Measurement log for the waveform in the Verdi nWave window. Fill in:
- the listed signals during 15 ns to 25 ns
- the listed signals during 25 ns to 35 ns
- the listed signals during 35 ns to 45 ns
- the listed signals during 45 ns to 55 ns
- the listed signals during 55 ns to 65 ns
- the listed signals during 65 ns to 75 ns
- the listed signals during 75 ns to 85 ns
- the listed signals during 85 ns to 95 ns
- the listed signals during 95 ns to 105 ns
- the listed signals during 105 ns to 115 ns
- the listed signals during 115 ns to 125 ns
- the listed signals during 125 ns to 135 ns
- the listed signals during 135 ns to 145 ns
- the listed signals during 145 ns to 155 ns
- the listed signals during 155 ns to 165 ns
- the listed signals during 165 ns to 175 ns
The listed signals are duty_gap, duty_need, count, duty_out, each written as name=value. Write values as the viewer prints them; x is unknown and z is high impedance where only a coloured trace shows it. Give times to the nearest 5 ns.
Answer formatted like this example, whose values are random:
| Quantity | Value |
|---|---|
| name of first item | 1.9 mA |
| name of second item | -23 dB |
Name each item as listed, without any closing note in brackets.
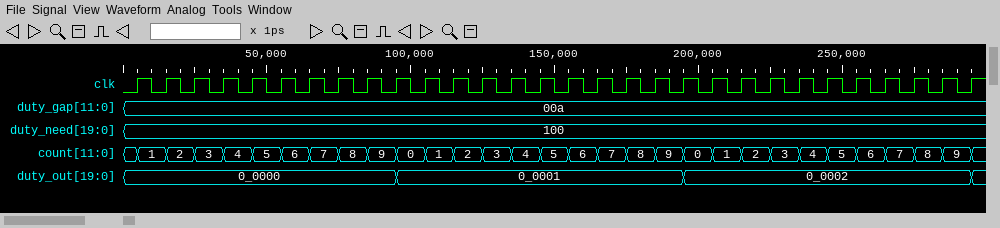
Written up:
| Quantity | Value |
|---|---|
| the listed signals during 15 ns to 25 ns | duty_gap=00a, duty_need=100, count=2, duty_out=0_0000 |
| the listed signals during 25 ns to 35 ns | duty_gap=00a, duty_need=100, count=3, duty_out=0_0000 |
| the listed signals during 35 ns to 45 ns | duty_gap=00a, duty_need=100, count=4, duty_out=0_0000 |
| the listed signals during 45 ns to 55 ns | duty_gap=00a, duty_need=100, count=5, duty_out=0_0000 |
| the listed signals during 55 ns to 65 ns | duty_gap=00a, duty_need=100, count=6, duty_out=0_0000 |
| the listed signals during 65 ns to 75 ns | duty_gap=00a, duty_need=100, count=7, duty_out=0_0000 |
| the listed signals during 75 ns to 85 ns | duty_gap=00a, duty_need=100, count=8, duty_out=0_0000 |
| the listed signals during 85 ns to 95 ns | duty_gap=00a, duty_need=100, count=9, duty_out=0_0000 |
| the listed signals during 95 ns to 105 ns | duty_gap=00a, duty_need=100, count=0, duty_out=0_0001 |
| the listed signals during 105 ns to 115 ns | duty_gap=00a, duty_need=100, count=1, duty_out=0_0001 |
| the listed signals during 115 ns to 125 ns | duty_gap=00a, duty_need=100, count=2, duty_out=0_0001 |
| the listed signals during 125 ns to 135 ns | duty_gap=00a, duty_need=100, count=3, duty_out=0_0001 |
| the listed signals during 135 ns to 145 ns | duty_gap=00a, duty_need=100, count=4, duty_out=0_0001 |
| the listed signals during 145 ns to 155 ns | duty_gap=00a, duty_need=100, count=5, duty_out=0_0001 |
| the listed signals during 155 ns to 165 ns | duty_gap=00a, duty_need=100, count=6, duty_out=0_0001 |
| the listed signals during 165 ns to 175 ns | duty_gap=00a, duty_need=100, count=7, duty_out=0_0001 |
